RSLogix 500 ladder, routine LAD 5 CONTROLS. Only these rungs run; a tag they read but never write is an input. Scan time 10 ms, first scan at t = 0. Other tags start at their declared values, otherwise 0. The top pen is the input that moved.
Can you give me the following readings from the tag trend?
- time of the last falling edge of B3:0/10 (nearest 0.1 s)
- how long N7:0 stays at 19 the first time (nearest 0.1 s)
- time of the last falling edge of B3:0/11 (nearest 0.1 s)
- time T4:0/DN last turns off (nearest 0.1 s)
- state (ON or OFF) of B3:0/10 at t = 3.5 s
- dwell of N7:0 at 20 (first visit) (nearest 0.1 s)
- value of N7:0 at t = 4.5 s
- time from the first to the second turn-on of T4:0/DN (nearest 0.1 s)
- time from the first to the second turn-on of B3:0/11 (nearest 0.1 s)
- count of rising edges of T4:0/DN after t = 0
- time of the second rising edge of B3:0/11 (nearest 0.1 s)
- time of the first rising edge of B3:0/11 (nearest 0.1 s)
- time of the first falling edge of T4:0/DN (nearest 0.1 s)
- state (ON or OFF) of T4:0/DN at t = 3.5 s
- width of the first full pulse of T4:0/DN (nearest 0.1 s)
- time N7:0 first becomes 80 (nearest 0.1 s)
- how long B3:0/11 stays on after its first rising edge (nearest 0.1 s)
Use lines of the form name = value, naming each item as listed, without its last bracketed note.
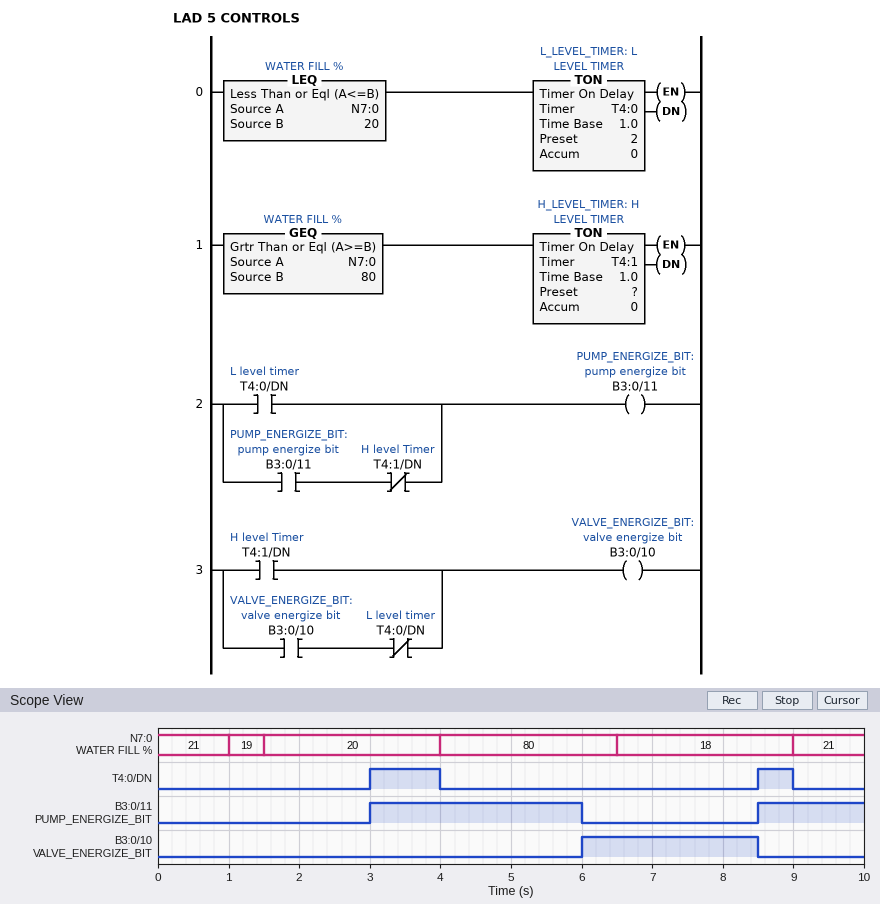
time of the last falling edge of B3:0/10 = 8.5 s
how long N7:0 stays at 19 the first time = 0.5 s
time of the last falling edge of B3:0/11 = 6.0 s
time T4:0/DN last turns off = 9.0 s
state (ON or OFF) of B3:0/10 at t = 3.5 s = OFF
dwell of N7:0 at 20 (first visit) = 2.5 s
value of N7:0 at t = 4.5 s = 80
time from the first to the second turn-on of T4:0/DN = 5.5 s
time from the first to the second turn-on of B3:0/11 = 5.5 s
count of rising edges of T4:0/DN after t = 0 = 2
time of the second rising edge of B3:0/11 = 8.5 s
time of the first rising edge of B3:0/11 = 3.0 s
time of the first falling edge of T4:0/DN = 4.0 s
state (ON or OFF) of T4:0/DN at t = 3.5 s = ON
width of the first full pulse of T4:0/DN = 1.0 s
time N7:0 first becomes 80 = 4.0 s
how long B3:0/11 stays on after its first rising edge = 3.0 s
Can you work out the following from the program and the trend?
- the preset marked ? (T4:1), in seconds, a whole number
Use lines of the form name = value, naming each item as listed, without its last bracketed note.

the preset marked ? (T4:1), in seconds, a whole number = 2 s
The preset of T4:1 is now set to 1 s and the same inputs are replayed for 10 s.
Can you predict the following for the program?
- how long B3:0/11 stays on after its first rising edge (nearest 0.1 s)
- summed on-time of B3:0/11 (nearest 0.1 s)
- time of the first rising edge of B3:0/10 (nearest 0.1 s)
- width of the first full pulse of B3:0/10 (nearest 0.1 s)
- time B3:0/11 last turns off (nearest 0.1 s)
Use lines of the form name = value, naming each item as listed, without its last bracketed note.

how long B3:0/11 stays on after its first rising edge = 2.0 s
summed on-time of B3:0/11 = 3.5 s
time of the first rising edge of B3:0/10 = 5.0 s
width of the first full pulse of B3:0/10 = 3.5 s
time B3:0/11 last turns off = 5.0 s
